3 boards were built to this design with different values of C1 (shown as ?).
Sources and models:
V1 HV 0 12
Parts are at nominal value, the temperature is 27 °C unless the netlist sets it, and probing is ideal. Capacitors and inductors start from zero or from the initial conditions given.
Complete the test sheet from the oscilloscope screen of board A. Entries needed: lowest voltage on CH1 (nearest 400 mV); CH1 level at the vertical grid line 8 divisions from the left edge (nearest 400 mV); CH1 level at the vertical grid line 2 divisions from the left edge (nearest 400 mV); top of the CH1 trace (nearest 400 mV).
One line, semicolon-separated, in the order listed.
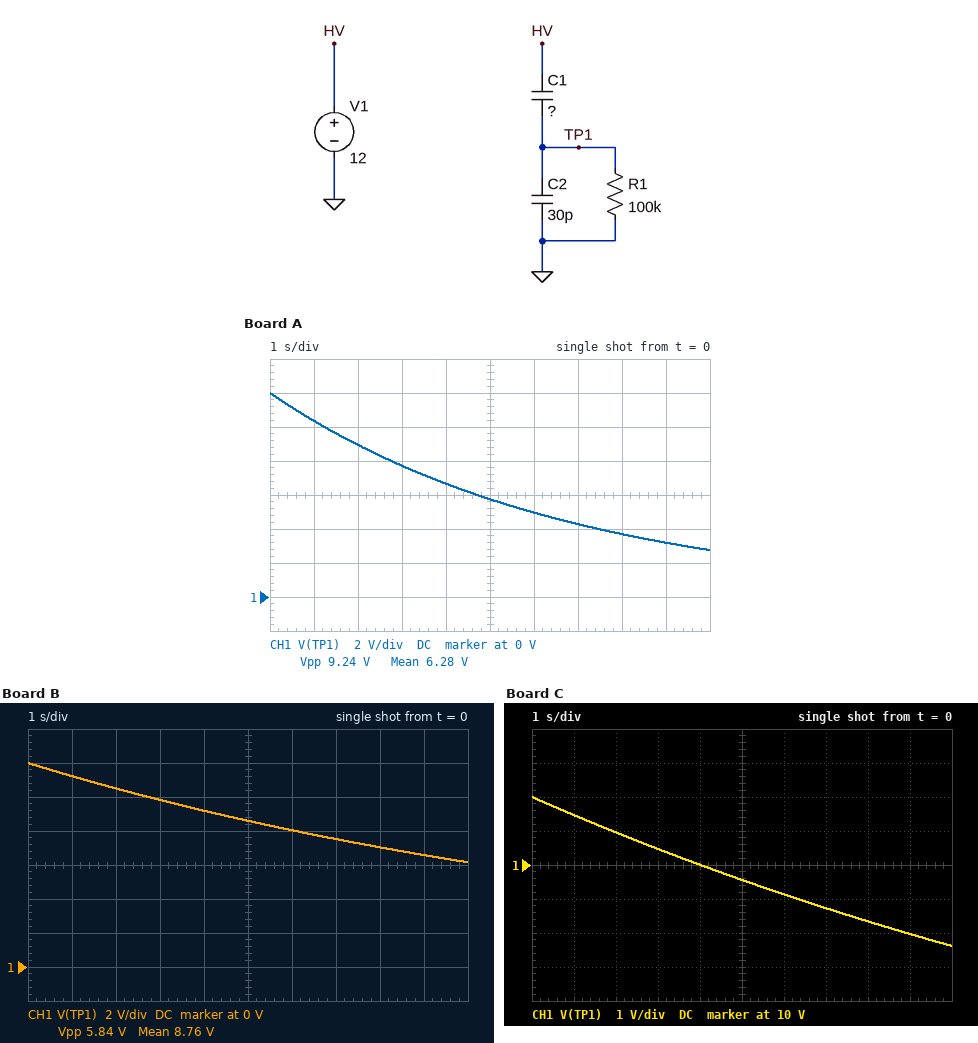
2.8 V; 3.6 V; 8.8 V; 12.0 V
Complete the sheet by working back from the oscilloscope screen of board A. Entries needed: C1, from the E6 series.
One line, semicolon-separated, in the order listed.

68 µF
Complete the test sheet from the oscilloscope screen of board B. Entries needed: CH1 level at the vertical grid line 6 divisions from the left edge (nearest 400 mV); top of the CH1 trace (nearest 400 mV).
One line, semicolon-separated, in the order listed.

8.0 V; 12.0 V
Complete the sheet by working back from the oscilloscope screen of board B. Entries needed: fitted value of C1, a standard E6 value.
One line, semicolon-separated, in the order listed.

150 µF
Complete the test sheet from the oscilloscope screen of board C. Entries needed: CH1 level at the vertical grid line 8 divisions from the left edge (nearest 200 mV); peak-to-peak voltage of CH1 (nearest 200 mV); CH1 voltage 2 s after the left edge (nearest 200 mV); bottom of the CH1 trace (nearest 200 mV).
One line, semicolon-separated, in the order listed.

8.4 V; 4.4 V; 11.0 V; 7.6 V
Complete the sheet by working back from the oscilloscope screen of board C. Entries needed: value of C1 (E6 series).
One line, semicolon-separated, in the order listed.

220 µF
